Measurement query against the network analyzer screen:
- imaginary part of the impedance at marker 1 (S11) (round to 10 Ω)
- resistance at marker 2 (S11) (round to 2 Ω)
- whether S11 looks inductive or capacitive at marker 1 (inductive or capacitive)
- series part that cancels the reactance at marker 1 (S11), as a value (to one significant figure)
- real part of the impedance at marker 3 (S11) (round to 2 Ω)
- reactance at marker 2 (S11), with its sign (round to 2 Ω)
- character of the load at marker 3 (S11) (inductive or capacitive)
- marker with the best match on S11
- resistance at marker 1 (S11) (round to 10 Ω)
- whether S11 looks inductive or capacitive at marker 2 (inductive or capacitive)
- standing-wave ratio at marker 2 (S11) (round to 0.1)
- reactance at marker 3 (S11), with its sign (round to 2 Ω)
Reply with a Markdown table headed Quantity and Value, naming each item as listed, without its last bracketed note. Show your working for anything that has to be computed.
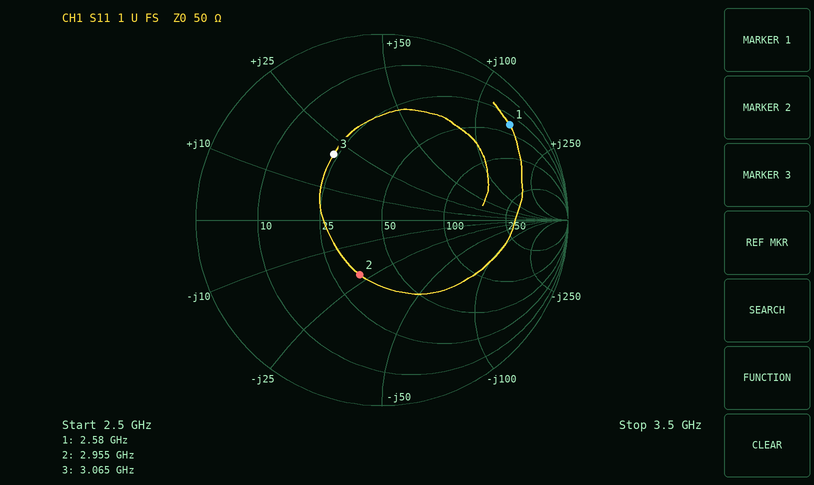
| Quantity | Value |
|---|---|
| imaginary part of the impedance at marker 1 (S11) | +140 Ω |
| resistance at marker 2 (S11) | 34 Ω |
| whether S11 looks inductive or capacitive at marker 1 | inductive |
| series part that cancels the reactance at marker 1 (S11), as a value | C = 1/(2π × 2.58 GHz × 140 Ω) ≈ 441 fF, so 400 fF to one significant figure |
| real part of the impedance at marker 3 (S11) | 24 Ω |
| reactance at marker 2 (S11), with its sign | -22 Ω |
| character of the load at marker 3 (S11) | inductive |
| marker with the best match on S11 | marker 2 |
| resistance at marker 1 (S11) | 40 Ω |
| whether S11 looks inductive or capacitive at marker 2 | capacitive |
| standing-wave ratio at marker 2 (S11) | 1.9 |
| reactance at marker 3 (S11), with its sign | +20 Ω |
